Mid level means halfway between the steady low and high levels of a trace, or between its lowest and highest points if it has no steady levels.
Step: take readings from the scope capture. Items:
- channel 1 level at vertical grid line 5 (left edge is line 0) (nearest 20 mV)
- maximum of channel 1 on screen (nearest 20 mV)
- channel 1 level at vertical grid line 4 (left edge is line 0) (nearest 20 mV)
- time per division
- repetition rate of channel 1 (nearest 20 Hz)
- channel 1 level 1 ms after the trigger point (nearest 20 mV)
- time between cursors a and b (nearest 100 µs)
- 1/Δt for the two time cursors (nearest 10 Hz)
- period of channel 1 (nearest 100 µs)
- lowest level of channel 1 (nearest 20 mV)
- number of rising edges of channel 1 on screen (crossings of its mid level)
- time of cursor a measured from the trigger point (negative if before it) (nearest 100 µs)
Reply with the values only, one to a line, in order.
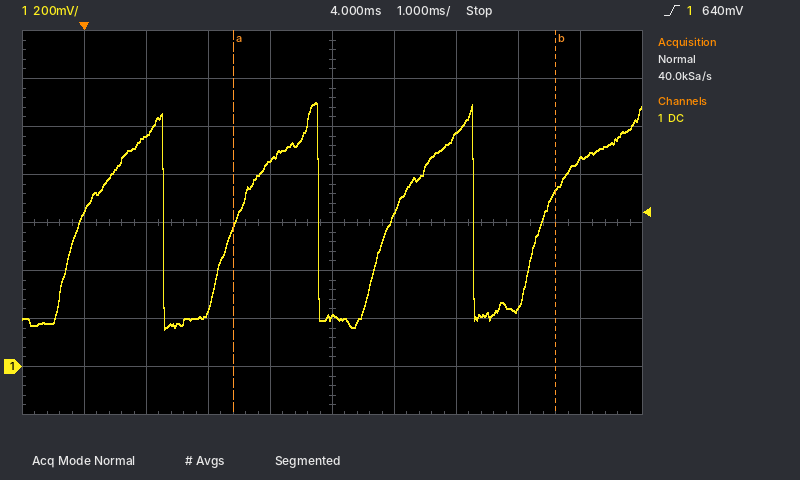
200 mV
1.10 V
860 mV
1 ms
400 Hz
960 mV
5.2 ms
190 Hz
2.5 ms
160 mV
4
+2.4 ms
